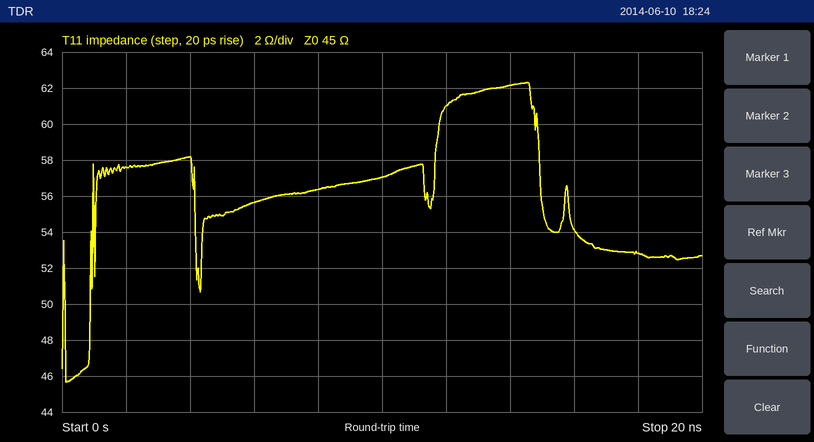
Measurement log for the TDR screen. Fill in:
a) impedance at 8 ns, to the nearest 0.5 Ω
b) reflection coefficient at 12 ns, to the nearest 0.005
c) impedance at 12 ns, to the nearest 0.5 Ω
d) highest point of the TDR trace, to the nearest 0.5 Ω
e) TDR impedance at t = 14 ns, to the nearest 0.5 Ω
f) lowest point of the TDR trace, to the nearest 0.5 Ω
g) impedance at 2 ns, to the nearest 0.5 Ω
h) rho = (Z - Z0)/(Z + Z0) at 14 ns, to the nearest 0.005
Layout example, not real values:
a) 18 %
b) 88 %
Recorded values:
a) 56.5 Ω
b) +0.150
c) 61.0 Ω
d) 62.5 Ω
e) 62.0 Ω
f) 45.5 Ω
g) 57.5 Ω
h) +0.160
